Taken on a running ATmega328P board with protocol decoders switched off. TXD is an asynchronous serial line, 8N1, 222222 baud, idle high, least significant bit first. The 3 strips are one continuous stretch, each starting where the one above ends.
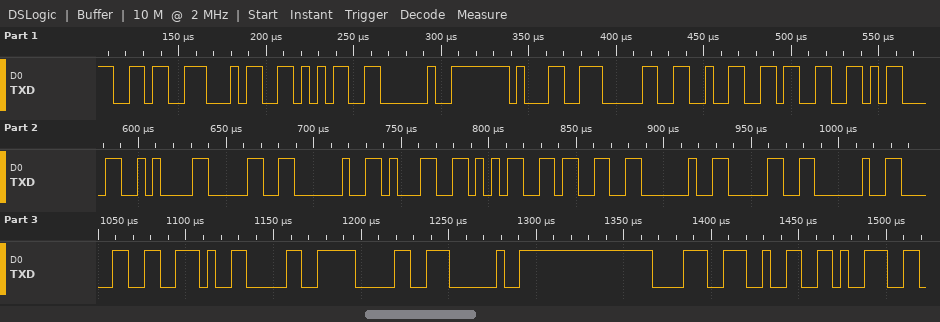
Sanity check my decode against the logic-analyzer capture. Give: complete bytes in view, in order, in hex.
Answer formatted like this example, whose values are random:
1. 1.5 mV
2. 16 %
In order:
1. 0x36 0x34 0x35 0x20 0x31 0x30 0x32 0x33 0x0D 0x0A 0x30 0x20 0x31 0x35 0x33 0x20 0x30 0x20 0x30 0x2E 0x30 0x30 0x20 0x38 0x32 0x39
